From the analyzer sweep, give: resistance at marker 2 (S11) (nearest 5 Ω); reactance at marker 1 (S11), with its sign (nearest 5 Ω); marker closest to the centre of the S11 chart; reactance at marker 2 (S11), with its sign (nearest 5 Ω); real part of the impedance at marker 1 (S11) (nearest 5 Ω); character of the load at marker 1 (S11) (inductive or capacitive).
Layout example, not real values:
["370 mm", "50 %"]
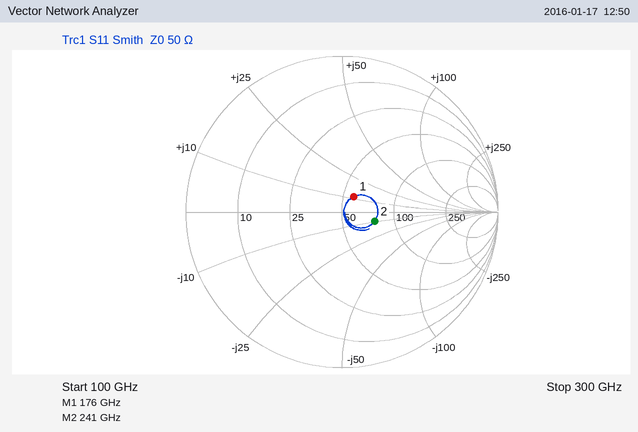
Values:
["75 Ω", "+10 Ω", "marker 1", "-10 Ω", "55 Ω", "inductive"]
